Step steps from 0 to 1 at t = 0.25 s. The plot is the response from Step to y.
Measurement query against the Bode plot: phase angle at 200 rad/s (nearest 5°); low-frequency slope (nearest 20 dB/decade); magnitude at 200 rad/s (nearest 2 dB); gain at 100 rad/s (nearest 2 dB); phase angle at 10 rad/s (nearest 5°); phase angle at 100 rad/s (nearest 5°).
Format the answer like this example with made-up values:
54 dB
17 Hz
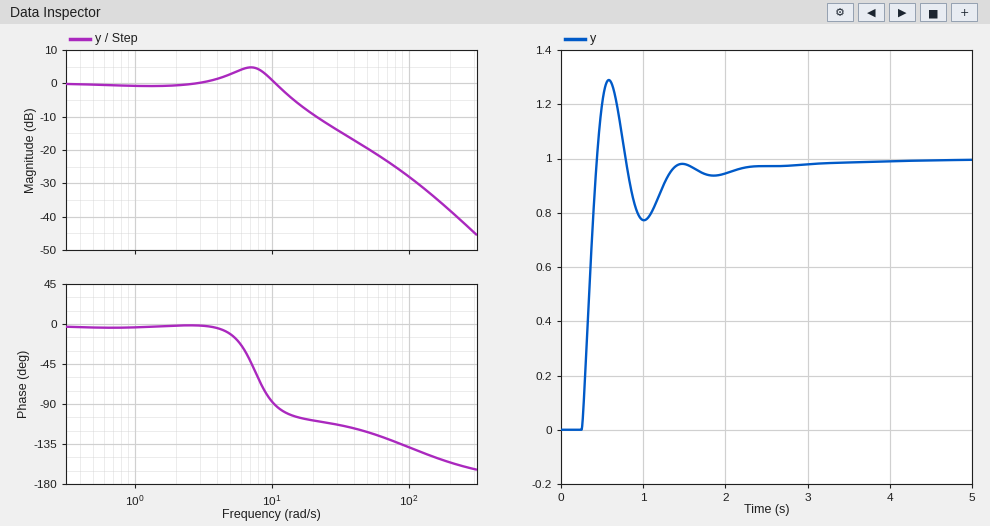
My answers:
-155°
0 dB/decade
-38 dB
-28 dB
-85°
-140°
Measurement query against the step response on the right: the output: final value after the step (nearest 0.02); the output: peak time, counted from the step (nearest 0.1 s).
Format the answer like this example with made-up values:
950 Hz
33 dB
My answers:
1.00
0.3 s
